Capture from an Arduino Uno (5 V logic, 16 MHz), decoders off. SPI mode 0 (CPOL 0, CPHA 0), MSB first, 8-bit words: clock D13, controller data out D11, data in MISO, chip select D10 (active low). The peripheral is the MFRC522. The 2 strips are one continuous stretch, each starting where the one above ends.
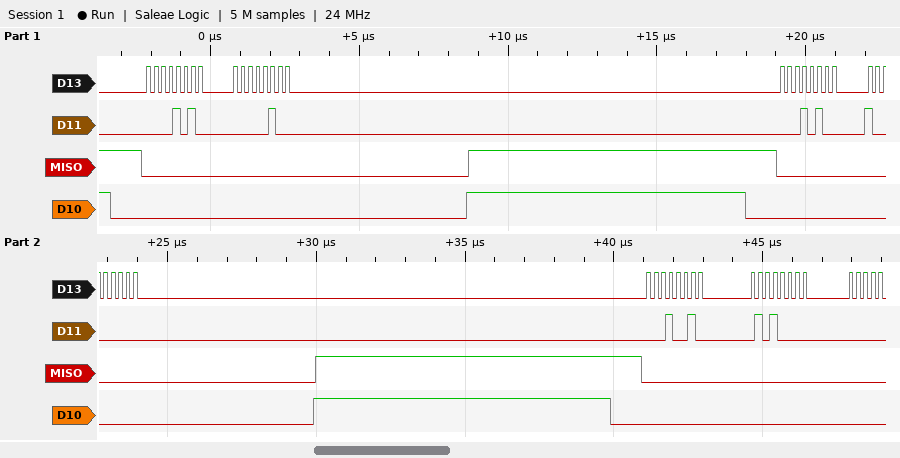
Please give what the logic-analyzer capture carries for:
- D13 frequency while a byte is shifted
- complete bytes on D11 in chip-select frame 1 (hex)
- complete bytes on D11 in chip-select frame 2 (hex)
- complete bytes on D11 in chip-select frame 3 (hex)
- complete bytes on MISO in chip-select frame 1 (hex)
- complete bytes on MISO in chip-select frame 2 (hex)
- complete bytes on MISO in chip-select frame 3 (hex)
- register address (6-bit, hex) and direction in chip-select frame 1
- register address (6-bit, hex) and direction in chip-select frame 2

4 MHz
0A 04
14 80
12 50
00 00
00 00
00 00
0x05 write
0x0A write
